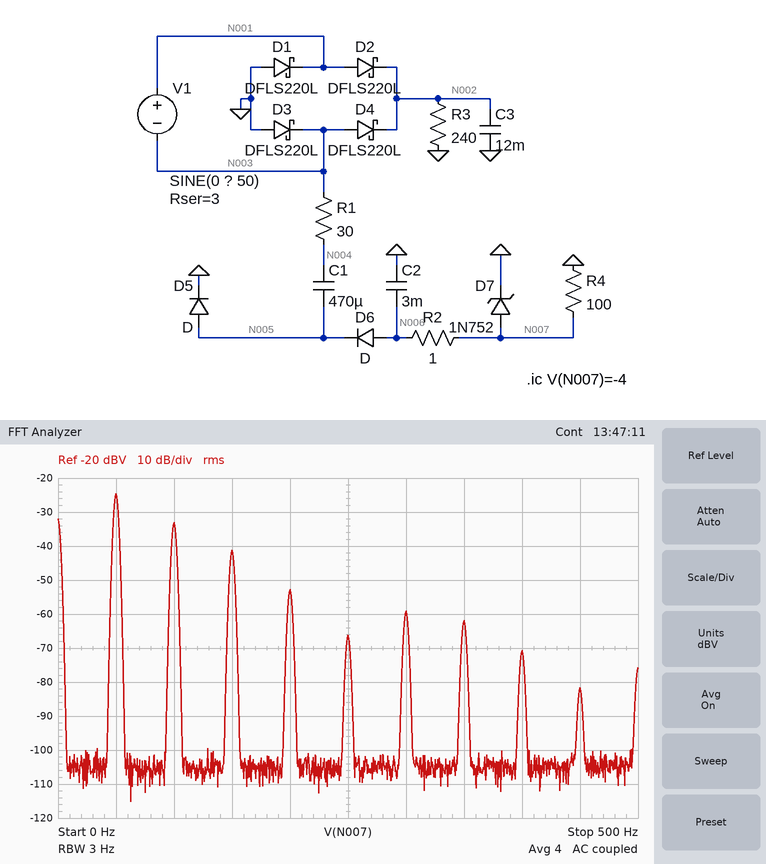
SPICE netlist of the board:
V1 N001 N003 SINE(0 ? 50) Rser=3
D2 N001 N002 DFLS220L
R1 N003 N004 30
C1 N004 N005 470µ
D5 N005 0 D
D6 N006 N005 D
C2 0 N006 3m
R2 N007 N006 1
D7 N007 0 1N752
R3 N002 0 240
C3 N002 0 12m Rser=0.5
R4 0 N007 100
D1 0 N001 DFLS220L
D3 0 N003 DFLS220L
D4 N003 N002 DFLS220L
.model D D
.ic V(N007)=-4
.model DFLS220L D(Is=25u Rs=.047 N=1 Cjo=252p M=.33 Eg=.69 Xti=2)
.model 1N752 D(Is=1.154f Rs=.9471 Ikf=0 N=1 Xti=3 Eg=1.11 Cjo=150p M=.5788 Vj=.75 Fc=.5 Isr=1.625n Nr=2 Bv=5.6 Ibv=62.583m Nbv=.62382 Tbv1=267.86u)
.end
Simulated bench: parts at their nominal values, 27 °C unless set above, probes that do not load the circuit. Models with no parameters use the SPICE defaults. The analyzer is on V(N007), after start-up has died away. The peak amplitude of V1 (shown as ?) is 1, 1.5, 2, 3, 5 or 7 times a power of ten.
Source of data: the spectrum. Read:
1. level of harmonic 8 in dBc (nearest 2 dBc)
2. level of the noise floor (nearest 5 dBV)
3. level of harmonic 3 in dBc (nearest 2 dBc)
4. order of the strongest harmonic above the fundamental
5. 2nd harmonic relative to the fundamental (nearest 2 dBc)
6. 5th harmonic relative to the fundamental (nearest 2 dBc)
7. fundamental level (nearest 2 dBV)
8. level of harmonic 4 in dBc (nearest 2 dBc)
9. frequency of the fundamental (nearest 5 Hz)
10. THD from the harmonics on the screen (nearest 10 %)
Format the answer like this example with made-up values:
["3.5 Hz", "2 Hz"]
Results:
["-46 dBc", "-105 dBV", "-16 dBc", "2", "-8 dBc", "-42 dBc", "-24 dBV", "-28 dBc", "50 Hz", "40 %"]
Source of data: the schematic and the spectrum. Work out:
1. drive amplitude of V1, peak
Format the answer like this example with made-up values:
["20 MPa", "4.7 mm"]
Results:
["20 V"]
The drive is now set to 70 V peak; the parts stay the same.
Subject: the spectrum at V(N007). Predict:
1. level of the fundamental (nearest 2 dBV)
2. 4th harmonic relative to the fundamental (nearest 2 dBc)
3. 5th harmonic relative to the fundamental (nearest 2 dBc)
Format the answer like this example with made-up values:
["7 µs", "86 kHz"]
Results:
["-18 dBV", "-36 dBc", "-32 dBc"]
